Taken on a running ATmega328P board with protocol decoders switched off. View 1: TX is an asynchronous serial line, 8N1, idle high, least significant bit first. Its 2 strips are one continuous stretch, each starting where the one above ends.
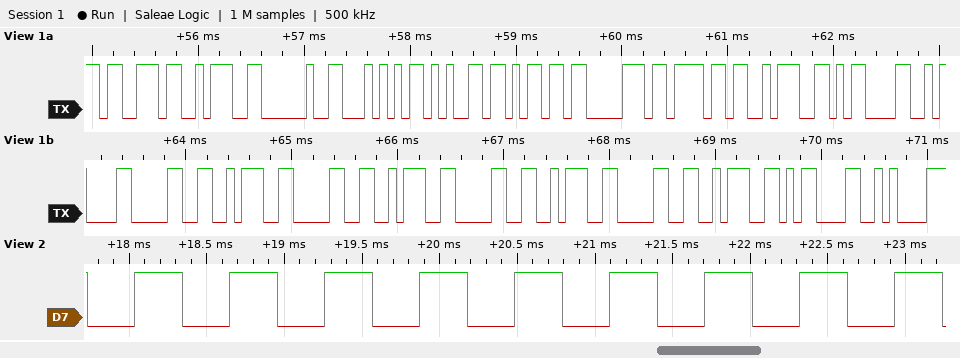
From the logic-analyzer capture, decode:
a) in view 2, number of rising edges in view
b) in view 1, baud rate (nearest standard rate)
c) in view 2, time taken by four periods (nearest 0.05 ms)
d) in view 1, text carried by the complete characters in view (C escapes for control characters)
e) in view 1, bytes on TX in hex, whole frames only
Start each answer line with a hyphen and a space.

- 9
- 14400 baud
- 2.45 ms
- "s: Tempo:\r\n0:0:0:0:\r\n"
- 73 3A 20 54 65 6D 70 6F 3A 0D 0A 30 3A 30 3A 30 3A 30 3A 0D 0A
